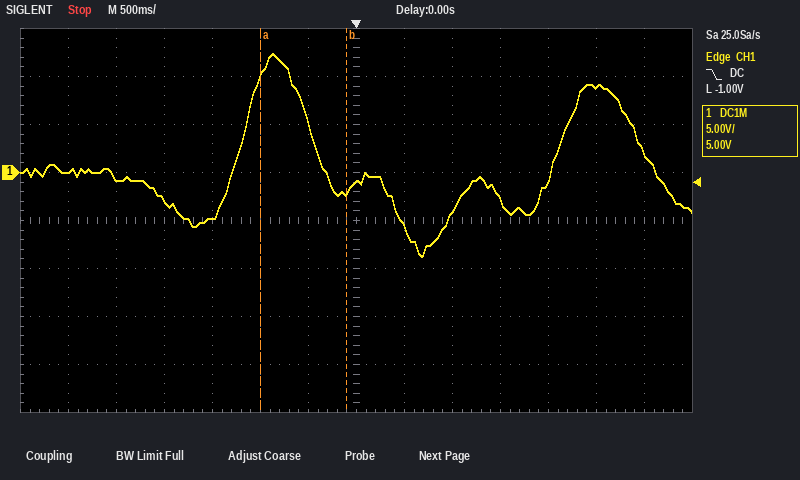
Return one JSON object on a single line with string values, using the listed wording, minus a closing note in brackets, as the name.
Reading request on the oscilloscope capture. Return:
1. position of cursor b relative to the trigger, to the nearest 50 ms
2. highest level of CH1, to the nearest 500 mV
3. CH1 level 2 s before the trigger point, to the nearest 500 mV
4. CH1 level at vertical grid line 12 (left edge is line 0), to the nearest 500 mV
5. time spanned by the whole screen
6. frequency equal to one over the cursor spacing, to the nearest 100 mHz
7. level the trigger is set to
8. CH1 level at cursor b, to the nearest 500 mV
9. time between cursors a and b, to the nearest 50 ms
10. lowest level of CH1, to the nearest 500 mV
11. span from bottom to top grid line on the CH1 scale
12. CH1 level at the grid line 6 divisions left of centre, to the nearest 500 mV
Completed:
{"position of cursor b relative to the trigger, to the nearest 50 ms": "-100 ms", "highest level of CH1, to the nearest 500 mV": "12.5 V", "CH1 level 2 s before the trigger point, to the nearest 500 mV": "-3.0 V", "CH1 level at vertical grid line 12 (left edge is line 0), to the nearest 500 mV": "9.0 V", "time spanned by the whole screen": "7 s", "frequency equal to one over the cursor spacing, to the nearest 100 mHz": "1.1 Hz", "level the trigger is set to": "-1.00 V", "CH1 level at cursor b, to the nearest 500 mV": "-2.0 V", "time between cursors a and b, to the nearest 50 ms": "900 ms", "lowest level of CH1, to the nearest 500 mV": "-9.0 V", "span from bottom to top grid line on the CH1 scale": "40 V", "CH1 level at the grid line 6 divisions left of centre, to the nearest 500 mV": "0.0 V"}
